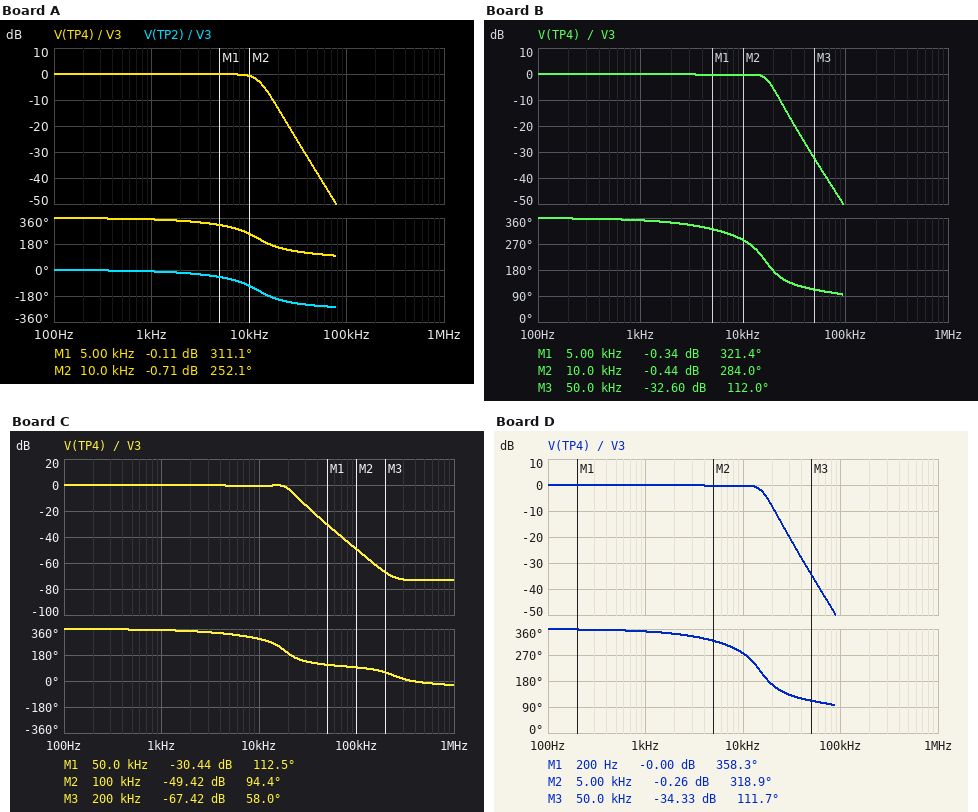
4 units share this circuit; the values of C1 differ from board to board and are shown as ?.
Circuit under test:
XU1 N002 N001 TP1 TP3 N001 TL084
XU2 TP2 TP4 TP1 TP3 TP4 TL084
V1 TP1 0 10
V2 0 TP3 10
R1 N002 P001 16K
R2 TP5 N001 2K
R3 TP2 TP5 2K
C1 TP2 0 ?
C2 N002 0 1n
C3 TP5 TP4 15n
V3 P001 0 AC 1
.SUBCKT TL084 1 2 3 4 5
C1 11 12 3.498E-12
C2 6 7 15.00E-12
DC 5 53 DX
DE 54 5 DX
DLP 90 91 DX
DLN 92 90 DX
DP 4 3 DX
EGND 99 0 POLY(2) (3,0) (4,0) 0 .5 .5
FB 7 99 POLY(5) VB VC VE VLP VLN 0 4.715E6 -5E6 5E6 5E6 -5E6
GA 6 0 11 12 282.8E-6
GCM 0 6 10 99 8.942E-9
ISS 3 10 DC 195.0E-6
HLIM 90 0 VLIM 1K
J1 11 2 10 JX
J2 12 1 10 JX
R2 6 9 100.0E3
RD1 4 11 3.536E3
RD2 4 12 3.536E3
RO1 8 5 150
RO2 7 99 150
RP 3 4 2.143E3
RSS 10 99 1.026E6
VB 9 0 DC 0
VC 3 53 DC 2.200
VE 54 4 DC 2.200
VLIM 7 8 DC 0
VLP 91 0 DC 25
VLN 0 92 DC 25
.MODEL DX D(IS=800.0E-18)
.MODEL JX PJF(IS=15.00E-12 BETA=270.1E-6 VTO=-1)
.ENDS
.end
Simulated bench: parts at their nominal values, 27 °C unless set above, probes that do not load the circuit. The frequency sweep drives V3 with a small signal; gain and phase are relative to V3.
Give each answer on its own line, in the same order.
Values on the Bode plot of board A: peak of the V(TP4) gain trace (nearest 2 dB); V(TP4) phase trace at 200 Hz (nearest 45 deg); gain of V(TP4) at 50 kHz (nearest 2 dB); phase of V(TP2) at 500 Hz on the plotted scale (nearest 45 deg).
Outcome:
0 dB
360 deg
-38 dB
0 deg
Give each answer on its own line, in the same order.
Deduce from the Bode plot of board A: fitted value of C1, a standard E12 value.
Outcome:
2.7 nF
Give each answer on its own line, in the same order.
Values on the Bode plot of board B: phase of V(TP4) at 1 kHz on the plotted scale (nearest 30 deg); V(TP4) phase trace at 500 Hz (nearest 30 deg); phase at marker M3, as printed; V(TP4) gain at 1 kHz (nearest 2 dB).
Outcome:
360 deg
360 deg
112.0 deg
0 dB
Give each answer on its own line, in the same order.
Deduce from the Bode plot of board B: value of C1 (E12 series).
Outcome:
1.5 nF
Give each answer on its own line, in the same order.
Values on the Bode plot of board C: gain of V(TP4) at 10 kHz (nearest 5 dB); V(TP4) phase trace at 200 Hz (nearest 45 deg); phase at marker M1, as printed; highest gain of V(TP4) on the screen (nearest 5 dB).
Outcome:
0 dB
360 deg
112.5 deg
0 dB
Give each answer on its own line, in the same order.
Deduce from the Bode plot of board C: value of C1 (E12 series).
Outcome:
1.2 nF
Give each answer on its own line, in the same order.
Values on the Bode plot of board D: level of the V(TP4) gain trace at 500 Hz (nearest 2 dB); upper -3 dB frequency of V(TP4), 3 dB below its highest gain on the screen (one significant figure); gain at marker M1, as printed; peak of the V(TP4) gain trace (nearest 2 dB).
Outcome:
0 dB
20 kHz
-0.00 dB
0 dB
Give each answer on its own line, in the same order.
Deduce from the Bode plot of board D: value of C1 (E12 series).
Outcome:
1.8 nF
